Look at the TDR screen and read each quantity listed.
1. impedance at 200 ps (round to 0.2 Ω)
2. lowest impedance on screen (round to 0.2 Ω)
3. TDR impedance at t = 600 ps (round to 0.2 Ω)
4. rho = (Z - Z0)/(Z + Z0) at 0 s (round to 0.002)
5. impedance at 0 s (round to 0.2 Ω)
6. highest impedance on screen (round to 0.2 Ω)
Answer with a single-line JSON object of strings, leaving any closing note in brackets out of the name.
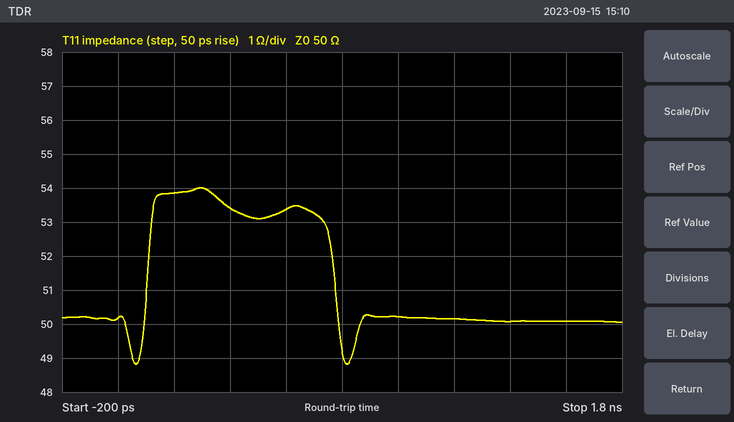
{"impedance at 200 ps": "53.8 Ω", "lowest impedance on screen": "48.8 Ω", "TDR impedance at t = 600 ps": "53.4 Ω", "rho = (Z - Z0)/(Z + Z0) at 0 s": "+0.002", "impedance at 0 s": "50.2 Ω", "highest impedance on screen": "54.0 Ω"}
